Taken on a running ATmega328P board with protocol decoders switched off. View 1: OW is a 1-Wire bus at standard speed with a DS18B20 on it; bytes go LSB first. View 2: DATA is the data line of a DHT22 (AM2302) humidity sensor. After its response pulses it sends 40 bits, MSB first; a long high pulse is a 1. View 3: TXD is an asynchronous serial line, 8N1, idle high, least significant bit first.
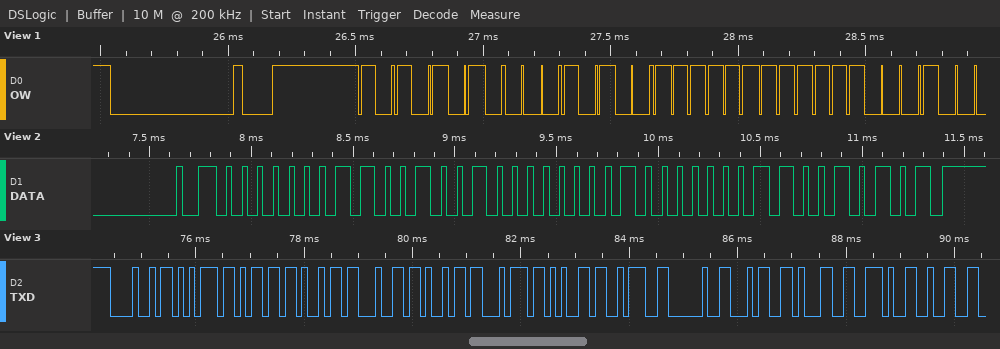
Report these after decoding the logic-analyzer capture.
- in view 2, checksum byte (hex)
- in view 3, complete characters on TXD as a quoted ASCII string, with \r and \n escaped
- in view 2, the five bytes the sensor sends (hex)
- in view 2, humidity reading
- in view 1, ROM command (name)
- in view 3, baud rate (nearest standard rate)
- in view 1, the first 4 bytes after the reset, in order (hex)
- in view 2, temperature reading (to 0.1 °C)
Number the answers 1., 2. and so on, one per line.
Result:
1. 0x95
2. "Humidite: 41.2"
3. 01 92 01 01 95
4. 40.2 %
5. Match ROM
6. 9600 baud
7. 55 28 FF 8F
8. 25.7 °C
